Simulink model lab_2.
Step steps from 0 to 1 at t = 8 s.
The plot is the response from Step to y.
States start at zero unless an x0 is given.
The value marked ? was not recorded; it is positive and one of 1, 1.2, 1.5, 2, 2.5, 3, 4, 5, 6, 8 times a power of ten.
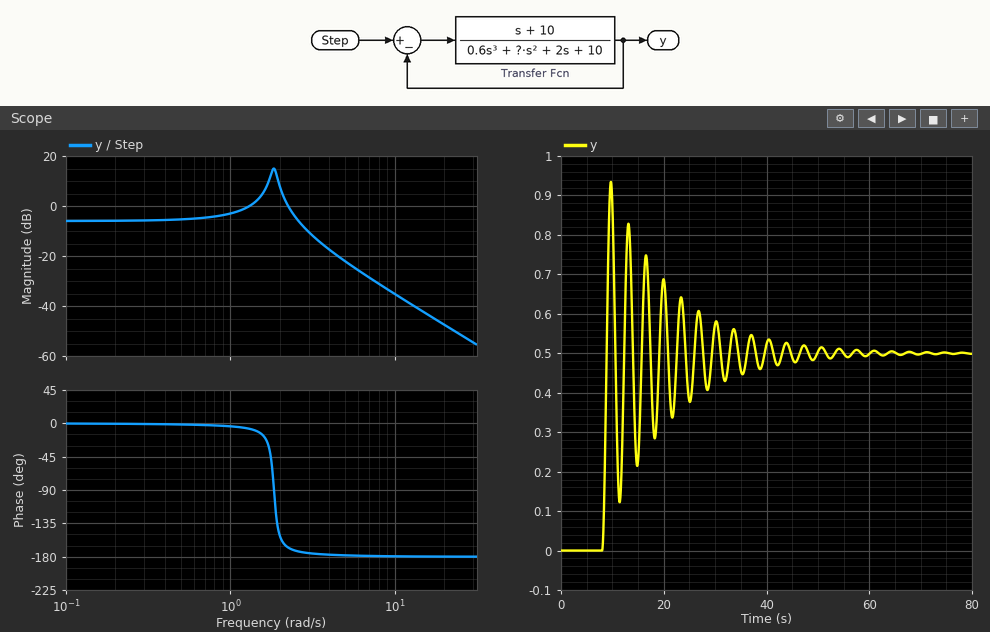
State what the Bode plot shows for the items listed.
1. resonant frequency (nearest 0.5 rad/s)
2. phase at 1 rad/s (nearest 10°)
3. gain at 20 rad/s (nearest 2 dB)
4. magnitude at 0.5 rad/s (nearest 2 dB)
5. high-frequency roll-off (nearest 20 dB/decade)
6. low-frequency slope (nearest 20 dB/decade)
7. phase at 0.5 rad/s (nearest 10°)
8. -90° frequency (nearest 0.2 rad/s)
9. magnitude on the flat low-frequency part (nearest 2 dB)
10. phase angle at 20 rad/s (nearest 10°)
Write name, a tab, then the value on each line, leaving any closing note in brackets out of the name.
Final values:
resonant frequency	2.0 rad/s
phase at 1 rad/s	0°
gain at 20 rad/s	-48 dB
magnitude at 0.5 rad/s	-6 dB
high-frequency roll-off	-40 dB/decade
low-frequency slope	0 dB/decade
phase at 0.5 rad/s	0°
-90° frequency	1.8 rad/s
magnitude on the flat low-frequency part	-6 dB
phase angle at 20 rad/s	-180°
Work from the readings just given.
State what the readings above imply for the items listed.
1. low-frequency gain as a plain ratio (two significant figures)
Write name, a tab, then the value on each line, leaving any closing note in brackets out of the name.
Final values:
low-frequency gain as a plain ratio	0.50
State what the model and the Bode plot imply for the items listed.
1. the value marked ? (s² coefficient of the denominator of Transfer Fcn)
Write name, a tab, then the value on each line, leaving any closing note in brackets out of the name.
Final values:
the value marked ?	6
